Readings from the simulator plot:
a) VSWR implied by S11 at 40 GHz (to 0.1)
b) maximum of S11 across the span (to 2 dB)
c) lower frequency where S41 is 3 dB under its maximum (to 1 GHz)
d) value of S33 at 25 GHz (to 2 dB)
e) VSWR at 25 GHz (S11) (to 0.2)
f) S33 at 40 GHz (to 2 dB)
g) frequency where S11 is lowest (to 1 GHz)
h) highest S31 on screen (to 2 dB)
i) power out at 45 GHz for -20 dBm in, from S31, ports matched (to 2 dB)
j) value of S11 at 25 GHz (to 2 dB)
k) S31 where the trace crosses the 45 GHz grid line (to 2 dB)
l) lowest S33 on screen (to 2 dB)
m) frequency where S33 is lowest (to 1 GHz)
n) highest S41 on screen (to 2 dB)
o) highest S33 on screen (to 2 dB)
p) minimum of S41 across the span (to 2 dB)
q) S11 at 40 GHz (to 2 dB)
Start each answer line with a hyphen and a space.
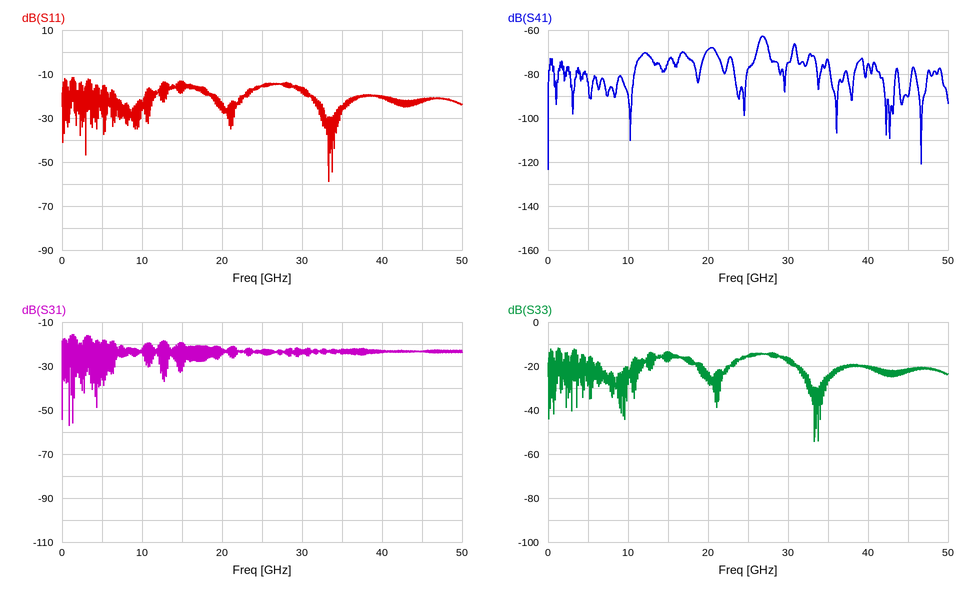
- 1.2
- -12 dB
- 26 GHz
- -16 dB
- 1.4
- -20 dB
- 33 GHz
- -16 dB
- -44 dBm
- -16 dB
- -24 dB
- -54 dB
- 33 GHz
- -62 dB
- -12 dB
- -124 dB
- -20 dB
